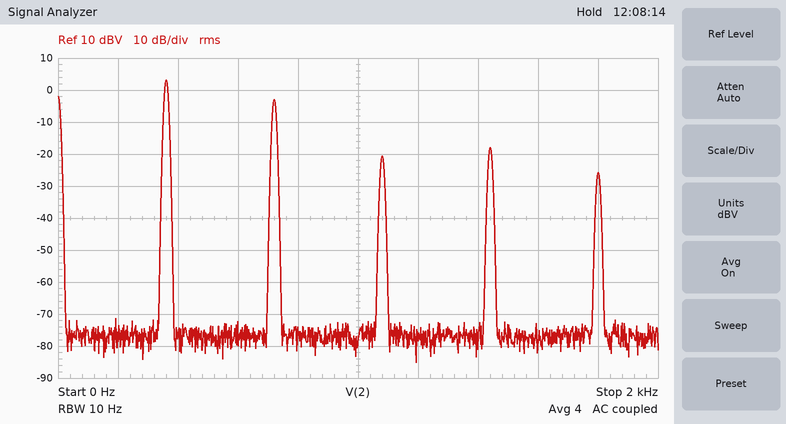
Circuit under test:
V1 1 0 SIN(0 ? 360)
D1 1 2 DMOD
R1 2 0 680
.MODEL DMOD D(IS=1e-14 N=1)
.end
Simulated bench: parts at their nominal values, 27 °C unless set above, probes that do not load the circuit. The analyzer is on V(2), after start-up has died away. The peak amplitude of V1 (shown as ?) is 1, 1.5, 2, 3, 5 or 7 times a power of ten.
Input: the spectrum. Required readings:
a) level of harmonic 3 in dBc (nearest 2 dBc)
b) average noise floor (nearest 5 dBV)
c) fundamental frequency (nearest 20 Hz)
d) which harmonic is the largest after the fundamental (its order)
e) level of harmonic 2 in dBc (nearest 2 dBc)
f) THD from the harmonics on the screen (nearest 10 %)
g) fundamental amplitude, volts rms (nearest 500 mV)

-24 dBc
-75 dBV
360 Hz
2
-6 dBc
50 %
1.5 V
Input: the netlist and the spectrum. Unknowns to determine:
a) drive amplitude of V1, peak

5 V
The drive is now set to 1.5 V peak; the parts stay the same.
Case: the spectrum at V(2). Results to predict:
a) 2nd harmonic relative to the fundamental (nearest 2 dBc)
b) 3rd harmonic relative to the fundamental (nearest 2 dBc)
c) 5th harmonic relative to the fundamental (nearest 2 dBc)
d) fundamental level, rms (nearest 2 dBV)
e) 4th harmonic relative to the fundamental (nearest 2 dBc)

-4 dBc
-12 dBc
-22 dBc
-12 dBV
-52 dBc
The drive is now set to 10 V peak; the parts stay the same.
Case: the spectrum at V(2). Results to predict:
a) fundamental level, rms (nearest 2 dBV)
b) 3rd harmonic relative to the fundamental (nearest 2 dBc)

10 dBV
-30 dBc
